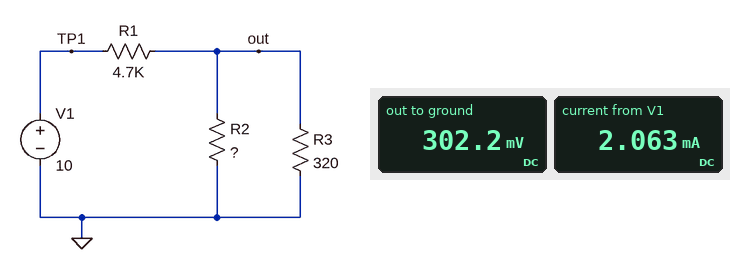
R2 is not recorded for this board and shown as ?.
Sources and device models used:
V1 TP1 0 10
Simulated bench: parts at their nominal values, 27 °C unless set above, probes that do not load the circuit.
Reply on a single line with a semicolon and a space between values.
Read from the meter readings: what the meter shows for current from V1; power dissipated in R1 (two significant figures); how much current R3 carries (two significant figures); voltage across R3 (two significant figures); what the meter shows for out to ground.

2.063 mA; 20 mW; 940 µA; 300 mV; 302.2 mV
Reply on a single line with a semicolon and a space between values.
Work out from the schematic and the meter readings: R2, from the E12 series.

270 Ω
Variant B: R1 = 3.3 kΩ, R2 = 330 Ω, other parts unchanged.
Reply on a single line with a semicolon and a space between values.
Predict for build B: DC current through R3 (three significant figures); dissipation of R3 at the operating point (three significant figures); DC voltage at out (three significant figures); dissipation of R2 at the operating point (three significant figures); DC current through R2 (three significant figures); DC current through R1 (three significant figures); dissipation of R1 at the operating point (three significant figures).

1.47 mA; 688 µW; 469 mV; 667 µW; 1.42 mA; 2.89 mA; 27.5 mW
